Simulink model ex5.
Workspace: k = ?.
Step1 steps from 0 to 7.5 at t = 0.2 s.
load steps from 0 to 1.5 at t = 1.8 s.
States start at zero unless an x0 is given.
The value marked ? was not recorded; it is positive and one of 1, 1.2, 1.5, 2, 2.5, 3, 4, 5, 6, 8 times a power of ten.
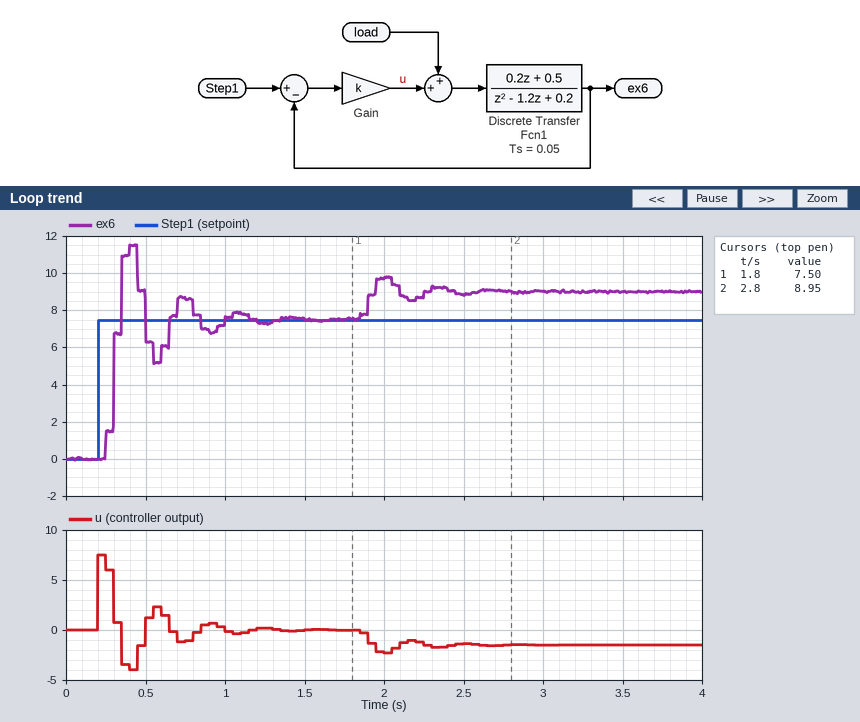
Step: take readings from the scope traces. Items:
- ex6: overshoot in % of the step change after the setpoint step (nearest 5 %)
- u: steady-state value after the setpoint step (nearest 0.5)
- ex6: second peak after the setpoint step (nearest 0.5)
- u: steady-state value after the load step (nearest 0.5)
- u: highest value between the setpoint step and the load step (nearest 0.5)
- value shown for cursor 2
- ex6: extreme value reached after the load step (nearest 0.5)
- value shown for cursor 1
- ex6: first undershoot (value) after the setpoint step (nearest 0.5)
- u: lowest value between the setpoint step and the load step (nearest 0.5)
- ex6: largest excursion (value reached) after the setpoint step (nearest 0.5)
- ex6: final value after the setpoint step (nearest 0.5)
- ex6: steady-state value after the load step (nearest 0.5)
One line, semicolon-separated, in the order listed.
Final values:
55 %; 0.0; 8.5; -1.5; 7.5; 8.95; 10.0; 7.50; 5.0; -4.0; 11.5; 7.5; 9.0
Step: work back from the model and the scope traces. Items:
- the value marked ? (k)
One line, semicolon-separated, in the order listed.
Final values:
1
